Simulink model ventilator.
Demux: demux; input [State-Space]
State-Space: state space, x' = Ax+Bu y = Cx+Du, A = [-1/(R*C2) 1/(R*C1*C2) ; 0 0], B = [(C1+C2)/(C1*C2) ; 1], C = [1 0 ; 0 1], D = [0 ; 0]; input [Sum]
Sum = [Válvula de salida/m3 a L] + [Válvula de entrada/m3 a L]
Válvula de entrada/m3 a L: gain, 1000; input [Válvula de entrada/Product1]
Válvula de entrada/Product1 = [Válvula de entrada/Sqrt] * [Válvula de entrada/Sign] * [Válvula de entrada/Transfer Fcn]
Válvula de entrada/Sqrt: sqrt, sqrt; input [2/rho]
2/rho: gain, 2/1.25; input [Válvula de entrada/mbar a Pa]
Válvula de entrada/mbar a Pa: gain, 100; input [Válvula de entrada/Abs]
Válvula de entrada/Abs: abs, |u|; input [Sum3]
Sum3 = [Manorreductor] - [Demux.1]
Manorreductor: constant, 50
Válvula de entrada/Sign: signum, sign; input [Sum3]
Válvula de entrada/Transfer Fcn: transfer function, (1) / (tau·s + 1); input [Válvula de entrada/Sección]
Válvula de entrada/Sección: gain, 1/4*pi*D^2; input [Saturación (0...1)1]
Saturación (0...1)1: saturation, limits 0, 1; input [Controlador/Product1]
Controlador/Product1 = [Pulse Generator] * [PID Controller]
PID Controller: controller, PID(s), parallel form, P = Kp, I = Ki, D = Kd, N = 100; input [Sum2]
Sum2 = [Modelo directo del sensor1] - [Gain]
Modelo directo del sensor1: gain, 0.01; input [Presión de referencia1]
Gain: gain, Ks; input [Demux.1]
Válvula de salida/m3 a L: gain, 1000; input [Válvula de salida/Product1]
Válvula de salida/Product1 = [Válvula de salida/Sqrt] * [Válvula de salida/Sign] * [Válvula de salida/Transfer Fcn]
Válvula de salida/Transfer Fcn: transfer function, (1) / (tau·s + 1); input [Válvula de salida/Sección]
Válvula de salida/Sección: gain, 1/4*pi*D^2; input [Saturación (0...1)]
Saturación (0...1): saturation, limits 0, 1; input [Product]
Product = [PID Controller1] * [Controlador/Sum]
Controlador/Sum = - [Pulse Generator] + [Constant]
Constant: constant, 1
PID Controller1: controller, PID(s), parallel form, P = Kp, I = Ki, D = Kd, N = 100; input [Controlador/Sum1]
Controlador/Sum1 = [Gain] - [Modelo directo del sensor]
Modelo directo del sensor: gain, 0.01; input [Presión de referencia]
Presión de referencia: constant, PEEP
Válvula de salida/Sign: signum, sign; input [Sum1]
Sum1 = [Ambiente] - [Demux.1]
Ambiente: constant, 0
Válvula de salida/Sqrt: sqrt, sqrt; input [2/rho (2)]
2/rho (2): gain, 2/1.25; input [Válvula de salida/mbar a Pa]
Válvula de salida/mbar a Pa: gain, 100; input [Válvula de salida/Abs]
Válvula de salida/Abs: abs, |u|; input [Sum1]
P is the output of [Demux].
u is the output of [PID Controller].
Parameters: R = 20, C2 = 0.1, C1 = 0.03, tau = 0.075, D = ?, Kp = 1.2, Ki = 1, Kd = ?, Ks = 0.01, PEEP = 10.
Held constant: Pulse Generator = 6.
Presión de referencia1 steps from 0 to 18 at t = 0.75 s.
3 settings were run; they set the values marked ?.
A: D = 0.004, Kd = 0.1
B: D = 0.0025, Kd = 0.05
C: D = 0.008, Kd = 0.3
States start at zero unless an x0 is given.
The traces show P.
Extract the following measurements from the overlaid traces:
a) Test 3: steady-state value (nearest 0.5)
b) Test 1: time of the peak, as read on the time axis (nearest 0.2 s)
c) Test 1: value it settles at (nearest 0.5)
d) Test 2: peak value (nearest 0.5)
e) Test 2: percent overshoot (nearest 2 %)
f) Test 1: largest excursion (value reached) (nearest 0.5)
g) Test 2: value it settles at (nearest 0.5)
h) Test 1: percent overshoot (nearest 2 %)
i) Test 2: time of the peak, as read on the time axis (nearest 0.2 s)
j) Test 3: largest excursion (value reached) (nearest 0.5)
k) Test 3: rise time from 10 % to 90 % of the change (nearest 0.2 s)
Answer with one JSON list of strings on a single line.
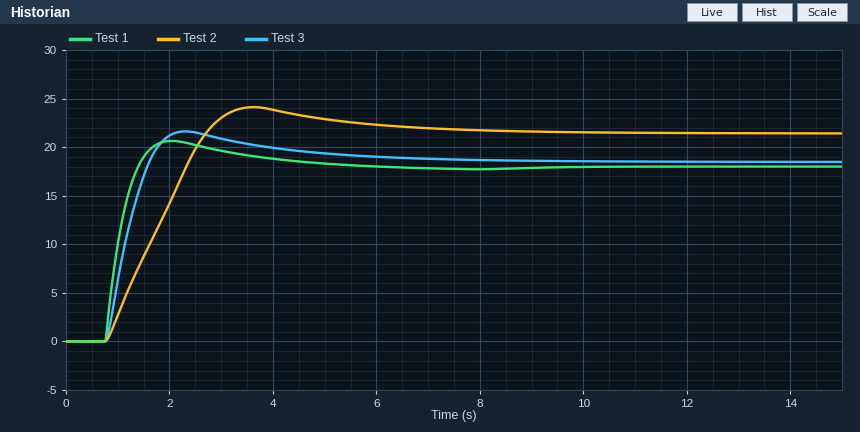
["18.5", "2.0 s", "18.0", "24.0", "12 %", "20.5", "21.5", "14 %", "3.6 s", "21.5", "0.6 s"]
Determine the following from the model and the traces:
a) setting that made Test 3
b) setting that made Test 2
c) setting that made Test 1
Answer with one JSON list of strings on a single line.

["A", "B", "C"]
